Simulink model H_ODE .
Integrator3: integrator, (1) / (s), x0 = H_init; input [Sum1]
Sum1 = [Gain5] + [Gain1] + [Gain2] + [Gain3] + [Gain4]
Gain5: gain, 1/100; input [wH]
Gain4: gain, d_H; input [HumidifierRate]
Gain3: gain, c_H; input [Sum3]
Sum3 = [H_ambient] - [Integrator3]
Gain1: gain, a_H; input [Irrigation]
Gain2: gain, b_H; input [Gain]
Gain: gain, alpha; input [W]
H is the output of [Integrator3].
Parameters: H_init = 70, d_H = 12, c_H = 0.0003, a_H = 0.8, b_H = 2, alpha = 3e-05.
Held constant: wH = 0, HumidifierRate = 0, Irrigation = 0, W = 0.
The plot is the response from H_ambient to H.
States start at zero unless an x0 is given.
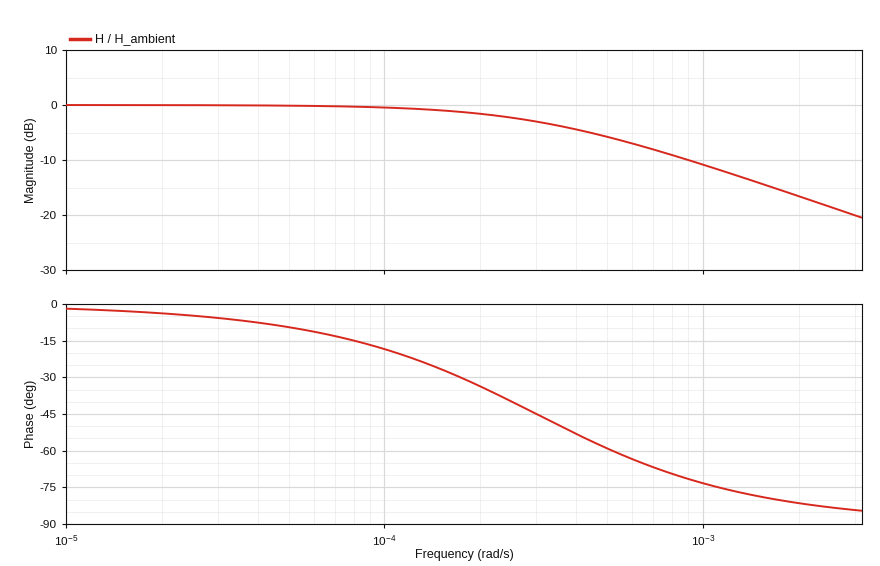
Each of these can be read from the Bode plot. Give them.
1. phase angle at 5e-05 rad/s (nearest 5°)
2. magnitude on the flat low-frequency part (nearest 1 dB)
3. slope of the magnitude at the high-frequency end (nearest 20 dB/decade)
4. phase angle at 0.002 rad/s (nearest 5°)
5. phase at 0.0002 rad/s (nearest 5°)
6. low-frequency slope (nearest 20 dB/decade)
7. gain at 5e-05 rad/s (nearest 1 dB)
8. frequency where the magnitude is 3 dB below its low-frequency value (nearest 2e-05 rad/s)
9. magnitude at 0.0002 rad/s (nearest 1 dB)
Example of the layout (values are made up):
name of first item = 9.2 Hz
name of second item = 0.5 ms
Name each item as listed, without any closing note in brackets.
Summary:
phase angle at 5e-05 rad/s = -10°
magnitude on the flat low-frequency part = 0 dB
slope of the magnitude at the high-frequency end = -20 dB/decade
phase angle at 0.002 rad/s = -80°
phase at 0.0002 rad/s = -35°
low-frequency slope = 0 dB/decade
gain at 5e-05 rad/s = 0 dB
frequency where the magnitude is 3 dB below its low-frequency value = 0.00030 rad/s
magnitude at 0.0002 rad/s = -2 dB
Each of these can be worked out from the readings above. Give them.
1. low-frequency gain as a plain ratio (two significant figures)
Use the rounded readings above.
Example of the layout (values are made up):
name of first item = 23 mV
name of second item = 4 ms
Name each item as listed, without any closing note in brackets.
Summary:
low-frequency gain as a plain ratio = 1.0
